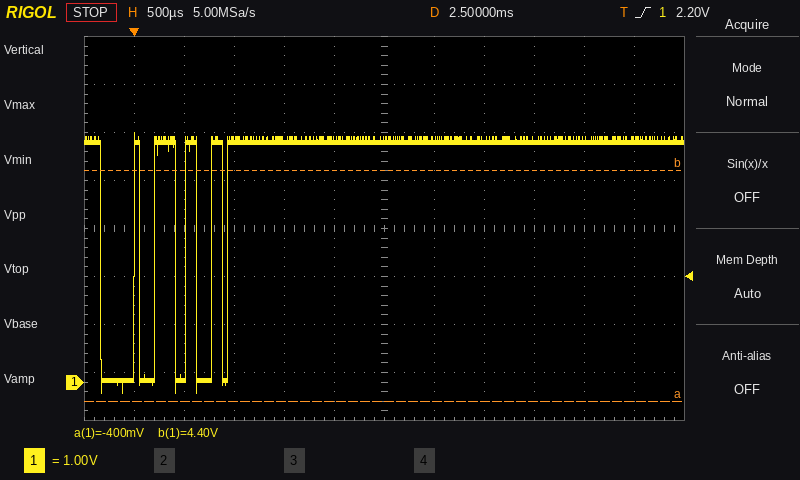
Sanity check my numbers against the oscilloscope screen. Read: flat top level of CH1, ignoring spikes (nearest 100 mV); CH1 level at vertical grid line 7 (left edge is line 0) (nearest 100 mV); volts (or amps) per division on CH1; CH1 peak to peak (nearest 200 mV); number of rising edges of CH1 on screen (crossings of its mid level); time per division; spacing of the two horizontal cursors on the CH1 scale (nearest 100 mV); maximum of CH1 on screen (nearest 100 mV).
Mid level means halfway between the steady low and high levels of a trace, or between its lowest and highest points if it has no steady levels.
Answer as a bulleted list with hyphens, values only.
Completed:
- 5.0 V
- 5.0 V
- 1 V
- 5.4 V
- 5
- 500 µs
- 4.8 V
- 5.2 V
